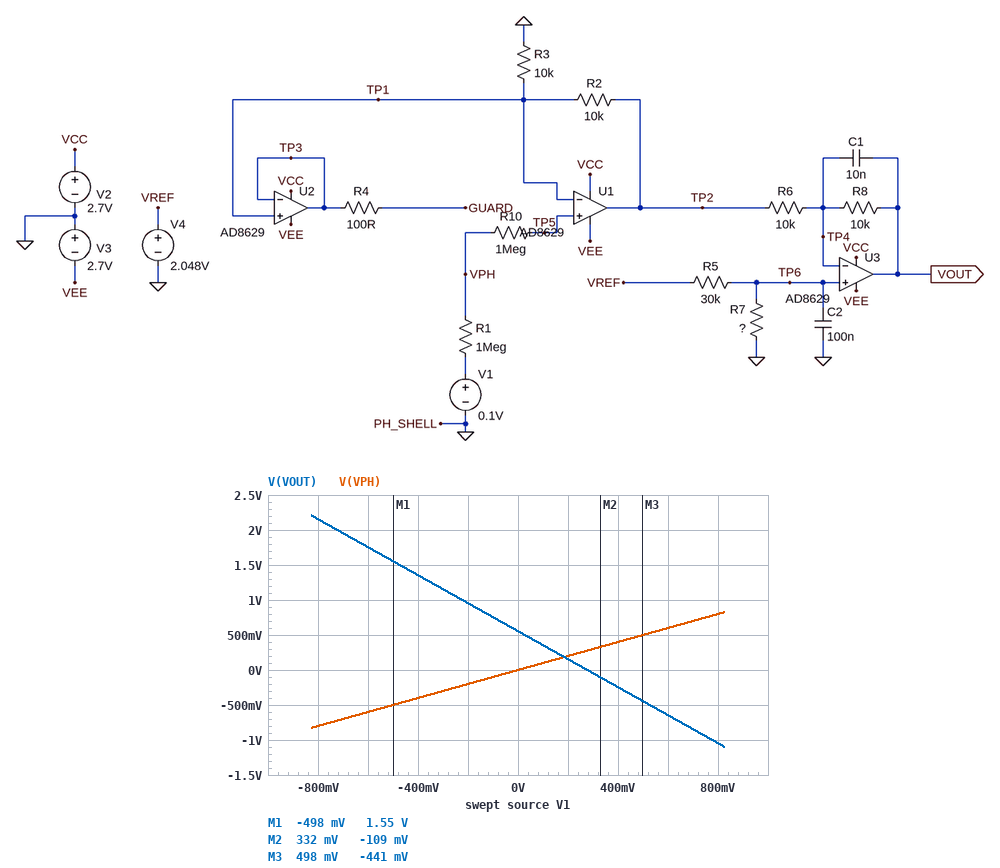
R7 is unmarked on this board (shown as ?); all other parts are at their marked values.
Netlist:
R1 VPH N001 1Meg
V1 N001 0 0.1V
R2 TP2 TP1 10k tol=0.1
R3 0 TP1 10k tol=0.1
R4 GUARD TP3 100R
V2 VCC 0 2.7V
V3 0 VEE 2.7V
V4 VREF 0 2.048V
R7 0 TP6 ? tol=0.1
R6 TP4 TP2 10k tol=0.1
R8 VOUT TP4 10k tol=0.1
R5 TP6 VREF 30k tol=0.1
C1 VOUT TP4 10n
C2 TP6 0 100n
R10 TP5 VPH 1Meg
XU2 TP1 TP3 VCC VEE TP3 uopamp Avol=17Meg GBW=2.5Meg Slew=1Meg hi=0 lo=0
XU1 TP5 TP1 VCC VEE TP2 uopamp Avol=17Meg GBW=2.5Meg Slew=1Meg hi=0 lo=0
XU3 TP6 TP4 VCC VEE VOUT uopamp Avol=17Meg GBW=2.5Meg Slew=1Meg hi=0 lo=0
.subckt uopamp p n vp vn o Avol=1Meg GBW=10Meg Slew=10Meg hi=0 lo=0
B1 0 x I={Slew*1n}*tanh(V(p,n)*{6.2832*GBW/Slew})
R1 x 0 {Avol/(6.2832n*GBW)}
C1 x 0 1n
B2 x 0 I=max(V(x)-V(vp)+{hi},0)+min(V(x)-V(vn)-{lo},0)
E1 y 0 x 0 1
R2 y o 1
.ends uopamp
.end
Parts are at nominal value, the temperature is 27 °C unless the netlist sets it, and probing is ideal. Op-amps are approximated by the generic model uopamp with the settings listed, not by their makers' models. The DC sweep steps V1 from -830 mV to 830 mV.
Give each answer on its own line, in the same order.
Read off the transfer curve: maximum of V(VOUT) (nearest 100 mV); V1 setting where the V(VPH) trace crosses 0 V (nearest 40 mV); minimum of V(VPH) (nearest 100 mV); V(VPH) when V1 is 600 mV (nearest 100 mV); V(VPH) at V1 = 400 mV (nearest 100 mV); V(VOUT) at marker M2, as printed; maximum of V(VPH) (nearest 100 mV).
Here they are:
2.2 V
0 V
-800 mV
600 mV
400 mV
-109 mV
800 mV
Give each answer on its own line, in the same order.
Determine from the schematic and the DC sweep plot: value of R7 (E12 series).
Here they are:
4.7 kΩ
